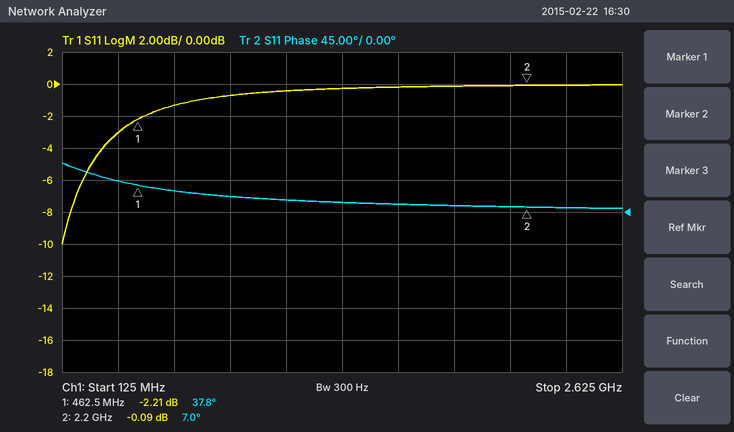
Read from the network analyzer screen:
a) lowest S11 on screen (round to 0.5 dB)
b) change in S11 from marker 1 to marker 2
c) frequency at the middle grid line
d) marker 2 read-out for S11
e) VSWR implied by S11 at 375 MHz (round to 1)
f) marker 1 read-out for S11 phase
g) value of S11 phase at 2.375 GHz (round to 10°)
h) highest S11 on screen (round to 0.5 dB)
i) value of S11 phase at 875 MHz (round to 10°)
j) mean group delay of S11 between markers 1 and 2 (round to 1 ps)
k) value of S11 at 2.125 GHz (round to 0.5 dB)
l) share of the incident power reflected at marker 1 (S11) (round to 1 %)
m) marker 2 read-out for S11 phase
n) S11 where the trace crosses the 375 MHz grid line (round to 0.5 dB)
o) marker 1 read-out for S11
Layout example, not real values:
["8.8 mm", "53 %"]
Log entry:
["-10.0 dB", "2.12 dB", "1.375 GHz", "-0.09 dB", "6", "37.8°", "10°", "0.0 dB", "20°", "49 ps", "0.0 dB", "60 %", "7.0°", "-3.0 dB", "-2.21 dB"]
